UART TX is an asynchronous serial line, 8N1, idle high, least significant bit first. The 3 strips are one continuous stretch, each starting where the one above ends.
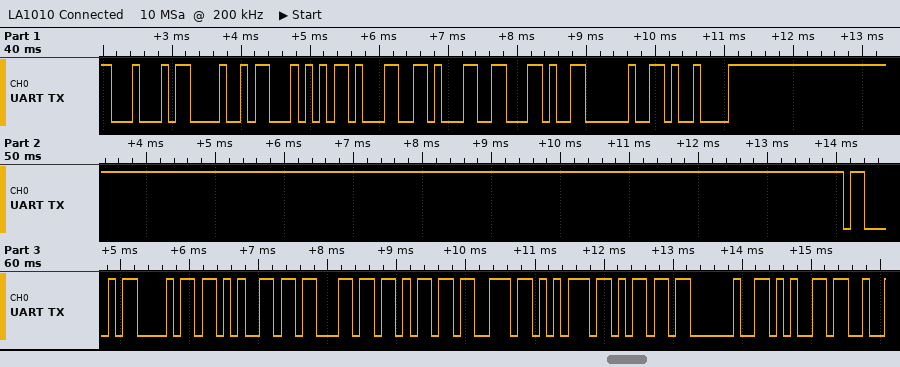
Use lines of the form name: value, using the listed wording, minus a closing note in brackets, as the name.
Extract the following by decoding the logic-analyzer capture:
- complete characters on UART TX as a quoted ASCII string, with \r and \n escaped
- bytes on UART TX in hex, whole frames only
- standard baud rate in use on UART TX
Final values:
complete characters on UART TX as a quoted ASCII string, with \r and \n escaped: "DHT11, \tChecksum e"
bytes on UART TX in hex, whole frames only: 44 48 54 31 31 2C 20 09 43 68 65 63 6B 73 75 6D 20 65
standard baud rate in use on UART TX: 9600 baud
